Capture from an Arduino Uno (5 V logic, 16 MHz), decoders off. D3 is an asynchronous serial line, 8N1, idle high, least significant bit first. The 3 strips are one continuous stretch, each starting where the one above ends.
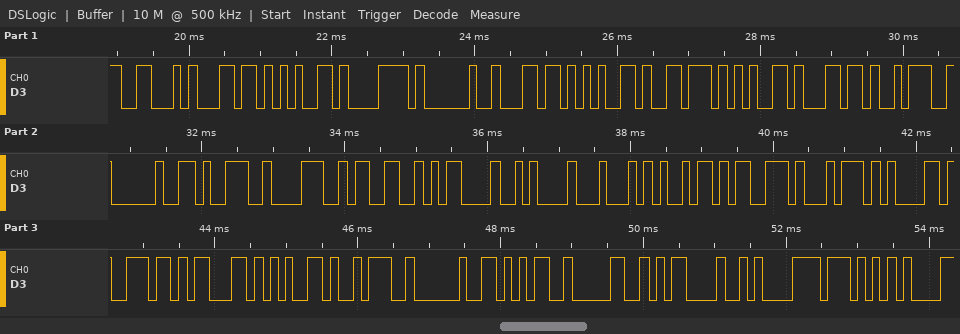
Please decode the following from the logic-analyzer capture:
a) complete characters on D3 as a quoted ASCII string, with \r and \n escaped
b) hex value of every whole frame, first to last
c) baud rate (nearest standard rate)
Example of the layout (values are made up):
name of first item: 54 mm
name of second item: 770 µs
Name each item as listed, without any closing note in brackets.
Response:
complete characters on D3 as a quoted ASCII string, with \r and \n escaped: "Flex level: 983\r\nDistance: 50\r\nW"
hex value of every whole frame, first to last: 0x46 0x6C 0x65 0x78 0x20 0x6C 0x65 0x76 0x65 0x6C 0x3A 0x20 0x39 0x38 0x33 0x0D 0x0A 0x44 0x69 0x73 0x74 0x61 0x6E 0x63 0x65 0x3A 0x20 0x35 0x30 0x0D 0x0A 0x57
baud rate: 9600 baud
